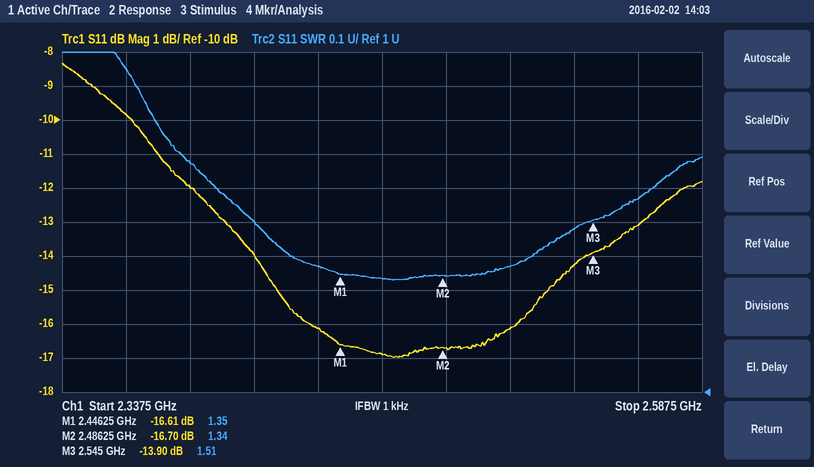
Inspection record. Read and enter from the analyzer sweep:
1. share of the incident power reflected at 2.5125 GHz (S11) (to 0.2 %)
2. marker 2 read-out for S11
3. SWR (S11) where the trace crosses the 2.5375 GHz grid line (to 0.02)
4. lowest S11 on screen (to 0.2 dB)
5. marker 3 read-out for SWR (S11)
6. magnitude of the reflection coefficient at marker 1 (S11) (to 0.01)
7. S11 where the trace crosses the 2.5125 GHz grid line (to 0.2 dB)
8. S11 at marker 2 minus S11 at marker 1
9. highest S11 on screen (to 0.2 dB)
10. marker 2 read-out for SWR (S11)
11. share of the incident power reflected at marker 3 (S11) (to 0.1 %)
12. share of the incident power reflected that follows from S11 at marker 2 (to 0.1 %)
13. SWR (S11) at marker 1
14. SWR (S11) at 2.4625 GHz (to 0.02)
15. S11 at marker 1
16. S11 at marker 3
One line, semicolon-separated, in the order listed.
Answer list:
2.4 %; -16.70 dB; 1.48; -17.0 dB; 1.51; 0.15; -16.2 dB; -0.09 dB; -8.4 dB; 1.34; 4.1 %; 2.1 %; 1.35; 1.34; -16.61 dB; -13.90 dB
